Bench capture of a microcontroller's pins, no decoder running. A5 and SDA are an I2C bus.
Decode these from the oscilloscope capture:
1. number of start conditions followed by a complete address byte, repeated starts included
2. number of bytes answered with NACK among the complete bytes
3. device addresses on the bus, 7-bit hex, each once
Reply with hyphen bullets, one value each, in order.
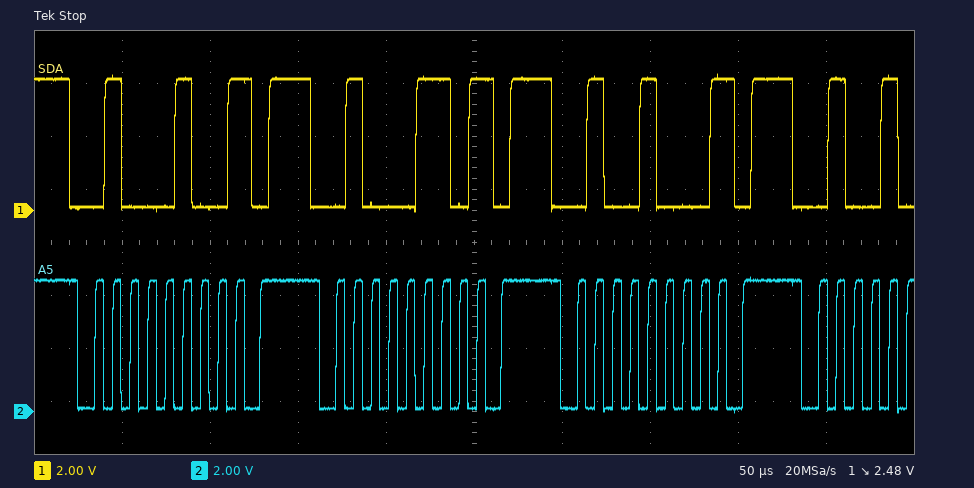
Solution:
- 3
- 3
- 0x22 0x23 0x24
